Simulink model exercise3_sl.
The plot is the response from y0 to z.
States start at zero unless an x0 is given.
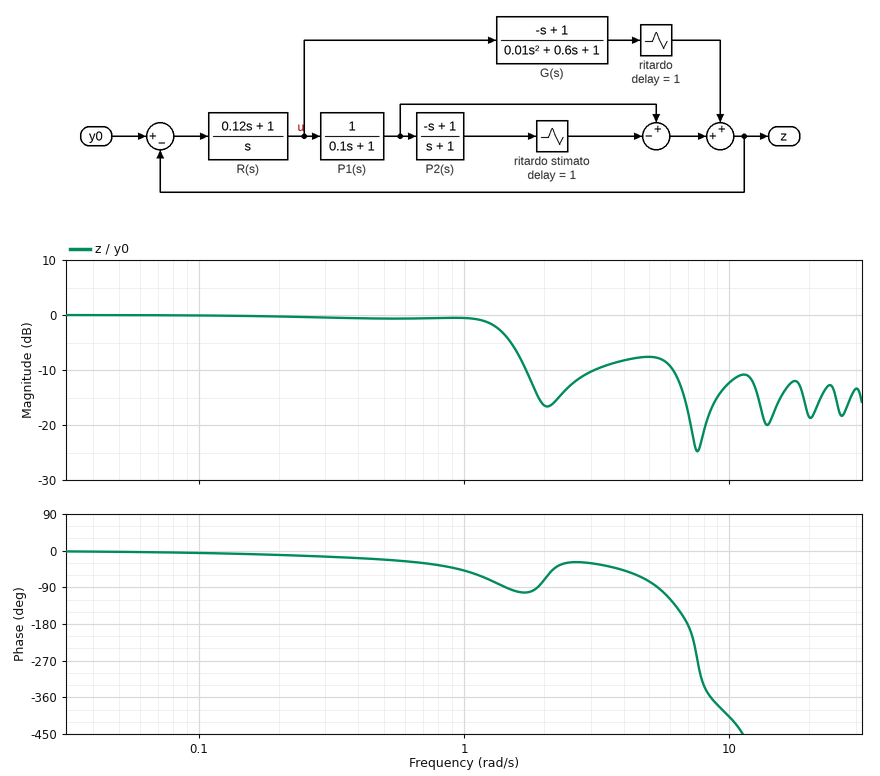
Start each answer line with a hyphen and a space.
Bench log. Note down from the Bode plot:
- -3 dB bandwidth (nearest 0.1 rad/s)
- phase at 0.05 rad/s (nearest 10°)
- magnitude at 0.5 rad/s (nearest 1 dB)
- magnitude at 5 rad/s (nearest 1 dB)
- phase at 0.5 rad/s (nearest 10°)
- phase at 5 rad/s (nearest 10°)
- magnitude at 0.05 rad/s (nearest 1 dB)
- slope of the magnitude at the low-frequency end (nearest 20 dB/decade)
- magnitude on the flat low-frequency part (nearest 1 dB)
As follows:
- 1.4 rad/s
- 0°
- -1 dB
- -8 dB
- -20°
- -80°
- 0 dB
- 0 dB/decade
- 0 dB
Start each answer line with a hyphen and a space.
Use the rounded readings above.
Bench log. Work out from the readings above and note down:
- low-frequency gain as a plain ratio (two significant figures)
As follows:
- 1.0
